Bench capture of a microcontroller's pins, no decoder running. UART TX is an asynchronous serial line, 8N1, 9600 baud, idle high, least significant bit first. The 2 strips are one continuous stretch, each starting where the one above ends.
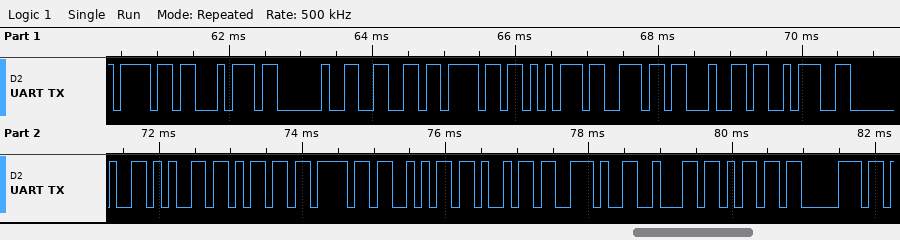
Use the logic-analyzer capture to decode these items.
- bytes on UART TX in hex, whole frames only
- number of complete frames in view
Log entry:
0x6F 0x74 0x20 0x66 0x6F 0x75 0x6E 0x64 0x3A 0x20 0x65 0x6D 0x6F 0x6A 0x69 0x2E 0x62 0x6D 0x70
19
